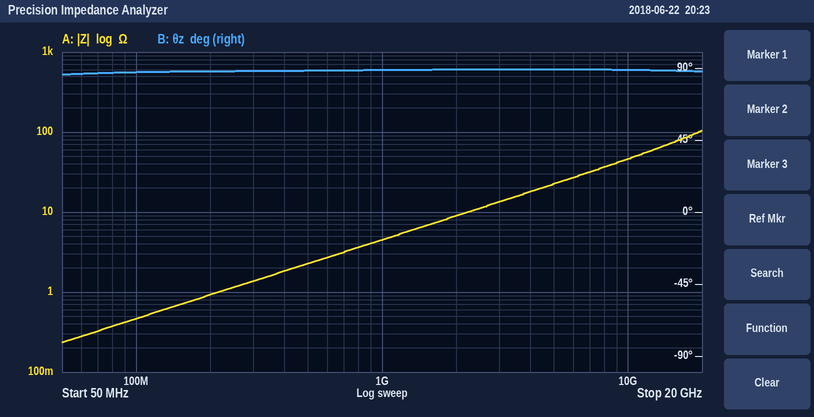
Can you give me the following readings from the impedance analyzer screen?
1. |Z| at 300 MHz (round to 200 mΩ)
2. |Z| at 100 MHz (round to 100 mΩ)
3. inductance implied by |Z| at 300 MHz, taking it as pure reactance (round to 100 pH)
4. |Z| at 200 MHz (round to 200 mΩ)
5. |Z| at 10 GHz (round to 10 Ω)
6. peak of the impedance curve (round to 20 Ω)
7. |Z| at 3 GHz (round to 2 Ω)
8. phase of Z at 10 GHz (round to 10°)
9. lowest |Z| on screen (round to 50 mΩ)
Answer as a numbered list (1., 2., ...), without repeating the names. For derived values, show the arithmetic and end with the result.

1. 1.4 Ω
2. 500 mΩ
3. L = 1.4 Ω/(2π × 300 MHz) ≈ 743 pH, so 700 pH to the nearest 100 pH
4. 1.0 Ω
5. 50 Ω
6. 100 Ω
7. 14 Ω
8. 90°
9. 250 mΩ
